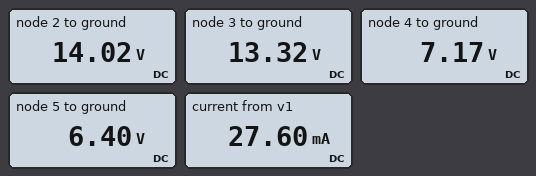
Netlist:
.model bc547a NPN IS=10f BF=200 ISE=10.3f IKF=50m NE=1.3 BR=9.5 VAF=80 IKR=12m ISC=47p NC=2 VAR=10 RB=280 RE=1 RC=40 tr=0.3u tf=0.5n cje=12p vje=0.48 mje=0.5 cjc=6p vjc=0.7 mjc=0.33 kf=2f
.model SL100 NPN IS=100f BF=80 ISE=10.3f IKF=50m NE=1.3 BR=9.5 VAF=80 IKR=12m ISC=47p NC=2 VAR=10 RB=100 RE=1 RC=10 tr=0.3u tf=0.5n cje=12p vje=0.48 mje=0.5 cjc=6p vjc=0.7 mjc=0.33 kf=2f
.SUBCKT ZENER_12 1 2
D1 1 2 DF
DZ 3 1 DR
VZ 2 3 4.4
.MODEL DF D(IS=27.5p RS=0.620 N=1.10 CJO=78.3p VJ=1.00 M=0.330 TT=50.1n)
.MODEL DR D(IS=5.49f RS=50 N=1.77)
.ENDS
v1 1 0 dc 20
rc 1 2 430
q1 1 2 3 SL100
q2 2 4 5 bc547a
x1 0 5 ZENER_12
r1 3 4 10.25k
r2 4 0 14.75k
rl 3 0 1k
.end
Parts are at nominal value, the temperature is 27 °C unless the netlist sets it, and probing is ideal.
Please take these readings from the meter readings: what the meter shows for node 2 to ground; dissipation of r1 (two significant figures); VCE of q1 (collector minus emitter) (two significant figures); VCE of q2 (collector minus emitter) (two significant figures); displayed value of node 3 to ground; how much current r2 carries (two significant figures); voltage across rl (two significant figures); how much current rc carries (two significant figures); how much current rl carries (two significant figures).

14.02 V
3.7 mW
6.7 V
7.6 V
13.32 V
490 µA
13 V
14 mA
13 mA
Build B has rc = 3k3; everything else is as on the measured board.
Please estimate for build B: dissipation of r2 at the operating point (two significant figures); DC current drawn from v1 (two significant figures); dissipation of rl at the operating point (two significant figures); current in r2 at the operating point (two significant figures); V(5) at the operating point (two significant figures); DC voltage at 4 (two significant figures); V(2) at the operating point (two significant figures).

2.8 mW
14 mA
120 mW
440 µA
5.7 V
6.4 V
12 V
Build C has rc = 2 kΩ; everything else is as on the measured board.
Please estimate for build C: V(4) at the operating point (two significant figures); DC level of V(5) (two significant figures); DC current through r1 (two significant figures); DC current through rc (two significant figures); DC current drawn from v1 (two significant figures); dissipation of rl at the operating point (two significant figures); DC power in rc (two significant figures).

6.5 V
5.8 V
470 µA
4.0 mA
16 mA
130 mW
31 mW
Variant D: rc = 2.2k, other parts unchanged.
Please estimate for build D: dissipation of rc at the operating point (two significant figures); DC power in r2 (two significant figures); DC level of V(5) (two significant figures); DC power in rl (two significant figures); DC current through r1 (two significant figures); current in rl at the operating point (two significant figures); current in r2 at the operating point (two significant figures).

29 mW
2.9 mW
5.8 V
130 mW
470 µA
11 mA
440 µA
